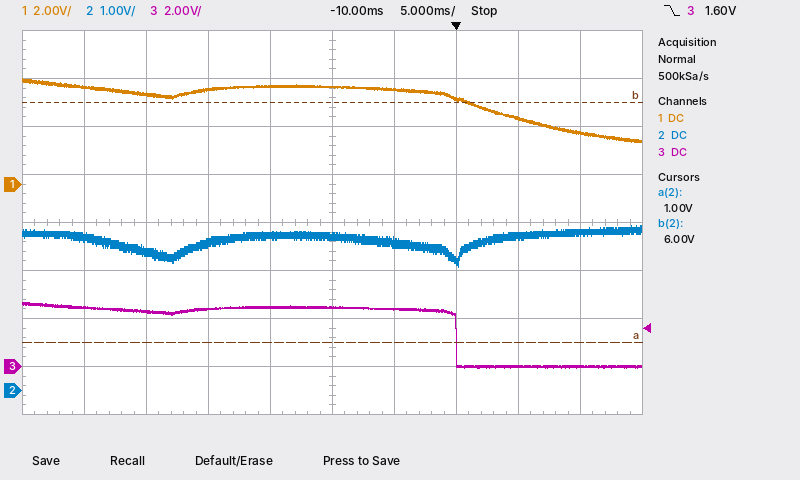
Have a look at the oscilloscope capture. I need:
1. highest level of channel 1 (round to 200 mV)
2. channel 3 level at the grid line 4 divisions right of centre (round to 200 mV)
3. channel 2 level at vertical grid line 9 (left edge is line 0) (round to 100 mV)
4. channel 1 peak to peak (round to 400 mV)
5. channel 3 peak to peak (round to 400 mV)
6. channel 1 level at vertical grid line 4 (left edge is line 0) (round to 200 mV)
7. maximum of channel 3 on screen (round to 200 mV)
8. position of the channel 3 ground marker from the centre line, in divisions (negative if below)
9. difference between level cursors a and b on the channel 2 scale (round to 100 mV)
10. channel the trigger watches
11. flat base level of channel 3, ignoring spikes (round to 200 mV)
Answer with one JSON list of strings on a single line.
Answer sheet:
["4.4 V", "0.0 V", "3.3 V", "2.8 V", "2.8 V", "4.0 V", "2.6 V", "-3.0 div", "5.0 V", "channel 3", "0.0 V"]
